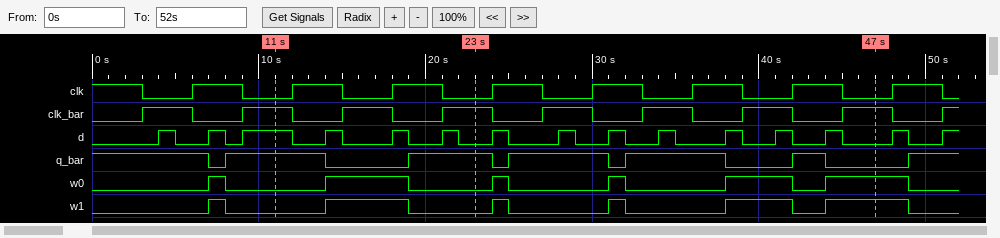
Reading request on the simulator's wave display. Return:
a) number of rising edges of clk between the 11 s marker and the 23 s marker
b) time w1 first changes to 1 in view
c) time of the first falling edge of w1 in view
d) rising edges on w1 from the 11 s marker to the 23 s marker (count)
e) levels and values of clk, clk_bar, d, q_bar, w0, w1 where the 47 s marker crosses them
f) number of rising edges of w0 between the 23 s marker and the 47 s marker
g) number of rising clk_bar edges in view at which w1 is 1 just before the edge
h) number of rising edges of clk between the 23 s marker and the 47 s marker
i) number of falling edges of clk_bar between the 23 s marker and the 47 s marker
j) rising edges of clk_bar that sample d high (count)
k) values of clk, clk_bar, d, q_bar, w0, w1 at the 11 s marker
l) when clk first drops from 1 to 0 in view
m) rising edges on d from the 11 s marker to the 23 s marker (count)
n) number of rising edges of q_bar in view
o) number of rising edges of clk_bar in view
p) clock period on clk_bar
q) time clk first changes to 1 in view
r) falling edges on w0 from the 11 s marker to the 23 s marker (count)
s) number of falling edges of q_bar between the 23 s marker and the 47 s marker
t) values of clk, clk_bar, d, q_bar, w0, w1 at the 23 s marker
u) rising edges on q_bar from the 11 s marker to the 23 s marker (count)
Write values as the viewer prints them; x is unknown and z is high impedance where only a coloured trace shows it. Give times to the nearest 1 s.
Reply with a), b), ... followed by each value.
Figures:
a) 2
b) 7 s
c) 8 s
d) 1
e) clk=0, clk_bar=1, d=0, q_bar=0, w0=1, w1=1
f) 4
g) 3
h) 4
i) 4
j) 3
k) clk=0, clk_bar=1, d=1, q_bar=1, w0=0, w1=0
l) 3 s
m) 3
n) 6
o) 9
p) 6 s
q) 6 s
r) 1
s) 4
t) clk=0, clk_bar=1, d=0, q_bar=1, w0=0, w1=0
u) 1
